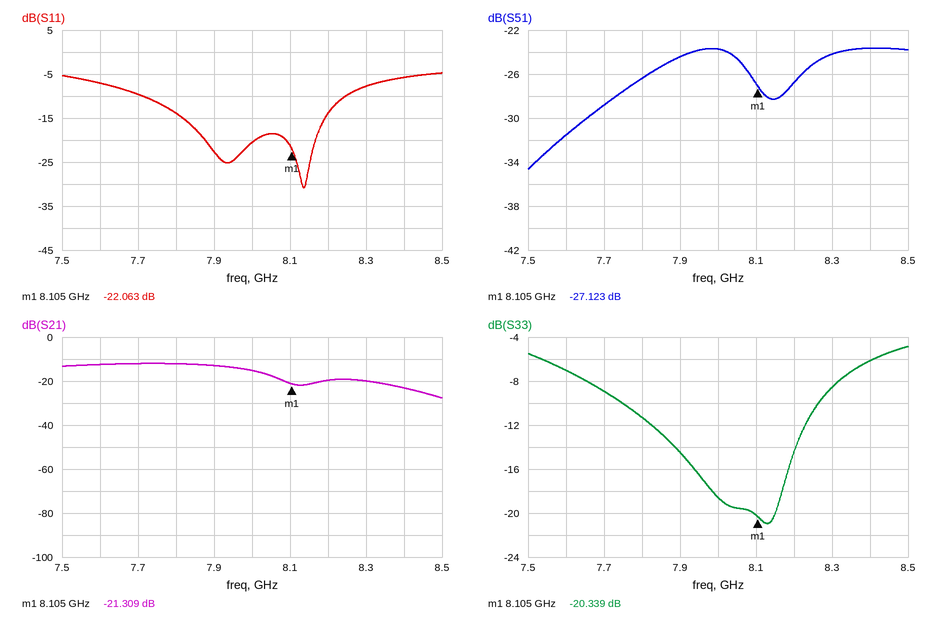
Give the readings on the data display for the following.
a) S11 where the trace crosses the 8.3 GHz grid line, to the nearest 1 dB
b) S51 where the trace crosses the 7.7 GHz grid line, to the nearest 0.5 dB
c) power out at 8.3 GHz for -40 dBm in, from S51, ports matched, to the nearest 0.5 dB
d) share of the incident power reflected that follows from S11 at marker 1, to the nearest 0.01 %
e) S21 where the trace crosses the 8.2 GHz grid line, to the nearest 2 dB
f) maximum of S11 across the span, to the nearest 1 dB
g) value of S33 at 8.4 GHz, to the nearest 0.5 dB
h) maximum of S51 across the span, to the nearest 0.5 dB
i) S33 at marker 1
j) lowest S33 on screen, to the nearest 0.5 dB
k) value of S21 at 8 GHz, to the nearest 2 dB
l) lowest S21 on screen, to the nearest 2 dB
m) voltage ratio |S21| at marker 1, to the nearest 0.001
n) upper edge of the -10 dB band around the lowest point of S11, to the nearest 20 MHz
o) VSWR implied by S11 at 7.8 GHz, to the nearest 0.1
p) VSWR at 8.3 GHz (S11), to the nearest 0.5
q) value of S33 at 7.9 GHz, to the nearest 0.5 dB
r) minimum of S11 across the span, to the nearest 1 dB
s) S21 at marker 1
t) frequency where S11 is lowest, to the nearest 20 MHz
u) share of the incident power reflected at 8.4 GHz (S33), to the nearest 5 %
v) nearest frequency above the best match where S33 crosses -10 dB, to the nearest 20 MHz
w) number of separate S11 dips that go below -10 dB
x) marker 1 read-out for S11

-8 dB
-29.0 dB
-64.0 dBm
0.62 %
-20 dB
-5 dB
-6.0 dB
-23.5 dB
-20.339 dB
-21.0 dB
-16 dB
-28 dB
0.086
8.24 GHz
1.5
2.5
-14.5 dB
-31 dB
-21.309 dB
8.14 GHz
25 %
8.26 GHz
2
-22.063 dB
